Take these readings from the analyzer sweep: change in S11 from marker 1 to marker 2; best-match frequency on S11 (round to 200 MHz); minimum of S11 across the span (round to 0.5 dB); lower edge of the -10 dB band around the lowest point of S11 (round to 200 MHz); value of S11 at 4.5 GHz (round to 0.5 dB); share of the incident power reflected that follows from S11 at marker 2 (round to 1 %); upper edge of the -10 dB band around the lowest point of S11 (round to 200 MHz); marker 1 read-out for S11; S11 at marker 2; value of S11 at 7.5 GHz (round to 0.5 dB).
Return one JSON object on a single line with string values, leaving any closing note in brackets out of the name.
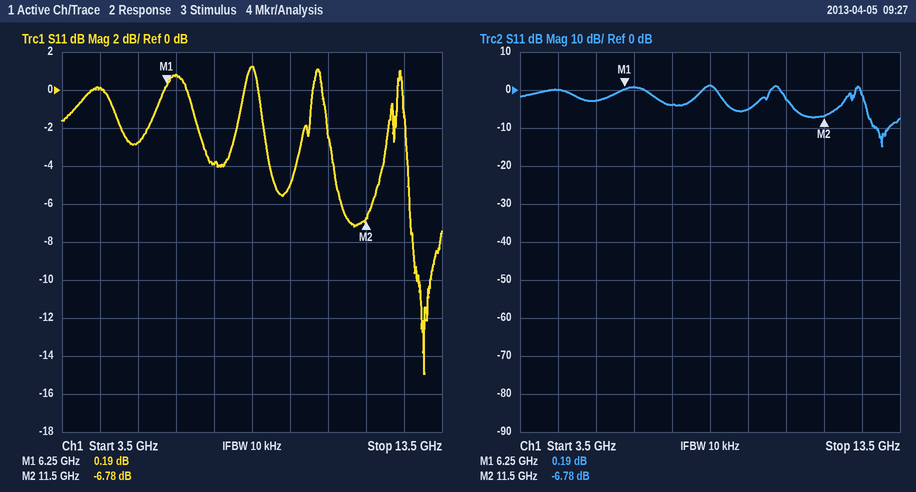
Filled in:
{"change in S11 from marker 1 to marker 2": "-6.97 dB", "best-match frequency on S11": "13.0 GHz", "minimum of S11 across the span": "-15.0 dB", "lower edge of the -10 dB band around the lowest point of S11": "12.8 GHz", "value of S11 at 4.5 GHz": "0.0 dB", "share of the incident power reflected that follows from S11 at marker 2": "21 %", "upper edge of the -10 dB band around the lowest point of S11": "13.2 GHz", "marker 1 read-out for S11": "0.19 dB", "S11 at marker 2": "-6.78 dB", "value of S11 at 7.5 GHz": "-4.0 dB"}
